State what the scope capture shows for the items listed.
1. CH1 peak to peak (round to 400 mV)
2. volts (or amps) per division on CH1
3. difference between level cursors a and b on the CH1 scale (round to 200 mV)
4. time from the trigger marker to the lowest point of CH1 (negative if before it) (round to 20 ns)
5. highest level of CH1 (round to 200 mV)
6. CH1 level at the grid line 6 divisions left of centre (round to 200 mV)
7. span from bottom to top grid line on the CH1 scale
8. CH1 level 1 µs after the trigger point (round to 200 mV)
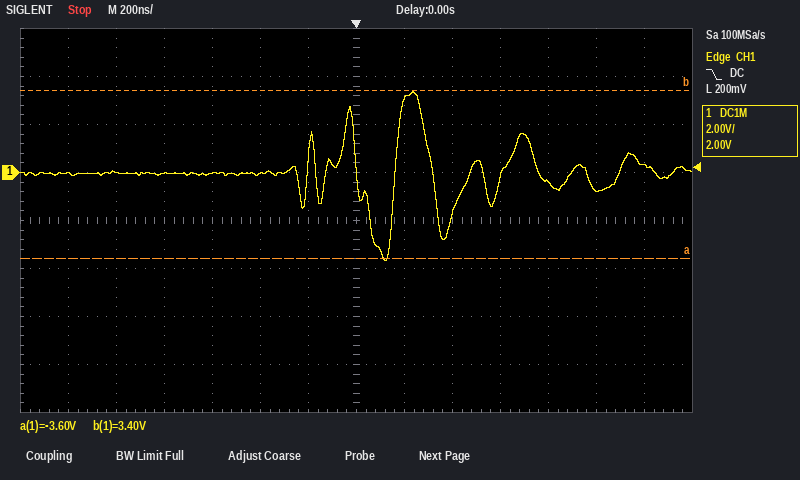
7.2 V
2 V
7.0 V
+120 ns
3.4 V
0.0 V
16 V
-800 mV
